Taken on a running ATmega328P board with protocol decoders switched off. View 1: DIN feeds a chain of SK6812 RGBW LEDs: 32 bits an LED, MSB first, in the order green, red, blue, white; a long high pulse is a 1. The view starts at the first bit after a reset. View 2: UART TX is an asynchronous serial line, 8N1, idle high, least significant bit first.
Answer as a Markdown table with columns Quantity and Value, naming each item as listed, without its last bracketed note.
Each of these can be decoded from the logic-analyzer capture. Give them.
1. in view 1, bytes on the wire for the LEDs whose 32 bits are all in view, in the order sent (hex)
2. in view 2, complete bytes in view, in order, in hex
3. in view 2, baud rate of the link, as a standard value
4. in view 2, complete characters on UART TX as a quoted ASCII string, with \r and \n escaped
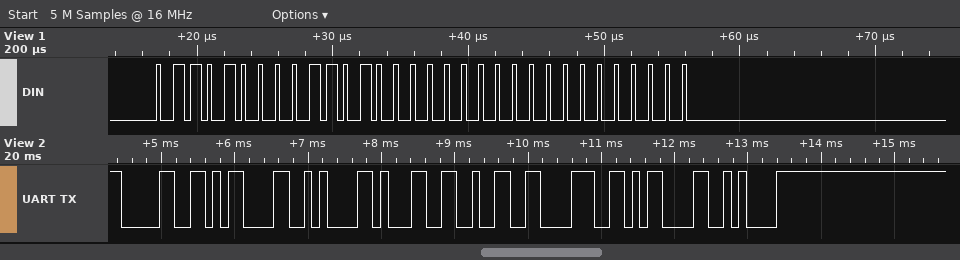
| Quantity | Value |
|---|---|
| in view 1, bytes on the wire for the LEDs whose 32 bits are all in view, in the order sent | 68 68 00 00 |
| in view 2, complete bytes in view, in order, in hex | 30 0D 0A 31 32 38 0D 0A |
| in view 2, baud rate of the link, as a standard value | 9600 baud |
| in view 2, complete characters on UART TX as a quoted ASCII string, with \r and \n escaped | "0\r\n128\r\n" |
